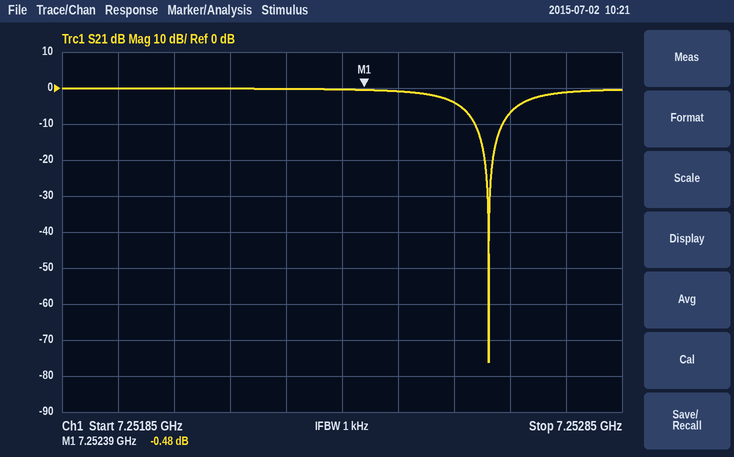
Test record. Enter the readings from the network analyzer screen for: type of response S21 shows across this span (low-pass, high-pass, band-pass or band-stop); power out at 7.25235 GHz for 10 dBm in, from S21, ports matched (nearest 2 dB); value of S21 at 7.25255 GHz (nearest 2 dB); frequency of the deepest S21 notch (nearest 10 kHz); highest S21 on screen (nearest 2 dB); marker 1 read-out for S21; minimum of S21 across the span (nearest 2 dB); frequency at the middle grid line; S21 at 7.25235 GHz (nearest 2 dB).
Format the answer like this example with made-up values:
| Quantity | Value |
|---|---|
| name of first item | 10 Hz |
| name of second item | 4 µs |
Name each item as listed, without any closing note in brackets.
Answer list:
| Quantity | Value |
|---|---|
| type of response S21 shows across this span | band-stop |
| power out at 7.25235 GHz for 10 dBm in, from S21, ports matched | 10 dBm |
| value of S21 at 7.25255 GHz | -4 dB |
| frequency of the deepest S21 notch | 7.25261 GHz |
| highest S21 on screen | 0 dB |
| marker 1 read-out for S21 | -0.48 dB |
| minimum of S21 across the span | -76 dB |
| frequency at the middle grid line | 7.25235 GHz |
| S21 at 7.25235 GHz | 0 dB |
